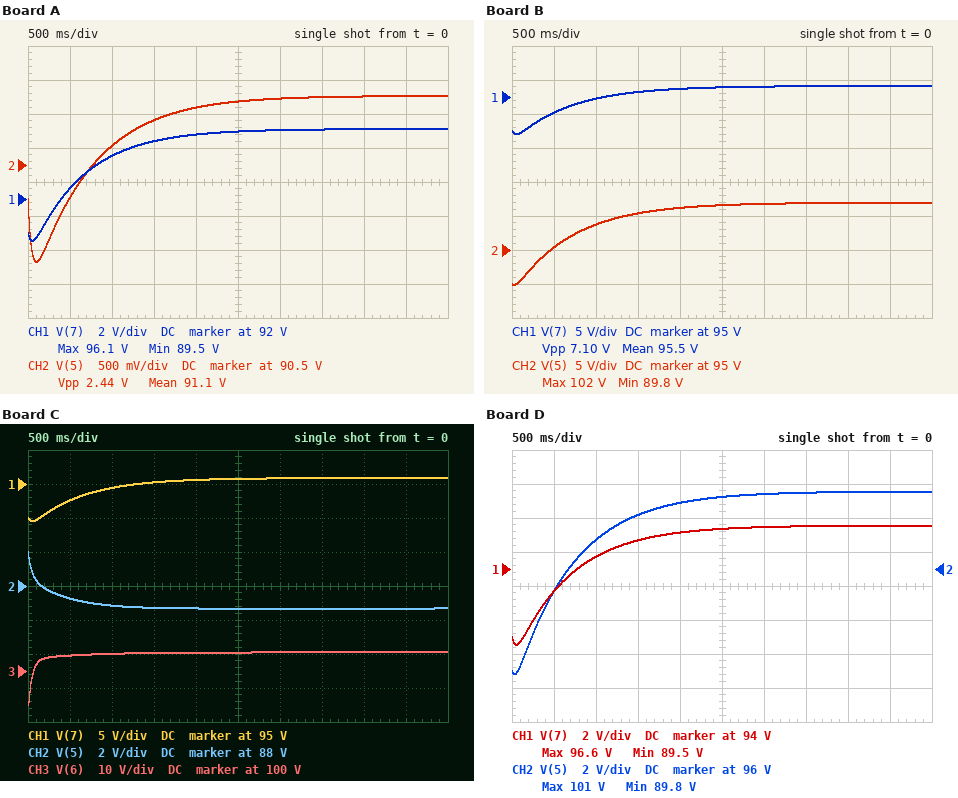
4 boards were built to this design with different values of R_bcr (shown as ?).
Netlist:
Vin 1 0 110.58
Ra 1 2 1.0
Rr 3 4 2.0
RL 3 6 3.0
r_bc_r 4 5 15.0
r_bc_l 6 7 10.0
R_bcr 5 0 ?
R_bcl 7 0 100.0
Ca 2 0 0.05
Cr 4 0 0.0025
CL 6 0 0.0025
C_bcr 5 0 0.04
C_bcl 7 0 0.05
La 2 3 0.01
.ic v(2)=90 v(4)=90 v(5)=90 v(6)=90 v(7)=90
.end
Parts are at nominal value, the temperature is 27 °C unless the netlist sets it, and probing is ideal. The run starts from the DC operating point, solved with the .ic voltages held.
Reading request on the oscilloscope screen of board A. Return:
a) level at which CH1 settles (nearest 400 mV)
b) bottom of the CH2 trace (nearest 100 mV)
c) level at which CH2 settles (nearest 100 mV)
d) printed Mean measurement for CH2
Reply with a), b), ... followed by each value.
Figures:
a) 96.0 V
b) 89.1 V
c) 91.5 V
d) 91.1 V
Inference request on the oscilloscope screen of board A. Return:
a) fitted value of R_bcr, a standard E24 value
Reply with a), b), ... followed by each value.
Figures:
a) 91 Ω
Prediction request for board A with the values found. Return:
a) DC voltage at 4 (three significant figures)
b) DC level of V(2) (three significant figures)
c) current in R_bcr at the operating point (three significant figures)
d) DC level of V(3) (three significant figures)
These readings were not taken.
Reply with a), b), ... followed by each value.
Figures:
a) 107 V
b) 109 V
c) 1.01 A
d) 109 V
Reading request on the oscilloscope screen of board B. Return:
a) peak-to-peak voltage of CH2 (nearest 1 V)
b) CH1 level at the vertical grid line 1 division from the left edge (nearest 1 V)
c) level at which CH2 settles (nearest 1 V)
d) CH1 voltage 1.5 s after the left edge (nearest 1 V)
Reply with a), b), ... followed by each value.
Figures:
a) 12 V
b) 93 V
c) 102 V
d) 96 V
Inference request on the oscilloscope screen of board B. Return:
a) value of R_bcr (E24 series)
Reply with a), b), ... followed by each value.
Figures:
a) 240 Ω
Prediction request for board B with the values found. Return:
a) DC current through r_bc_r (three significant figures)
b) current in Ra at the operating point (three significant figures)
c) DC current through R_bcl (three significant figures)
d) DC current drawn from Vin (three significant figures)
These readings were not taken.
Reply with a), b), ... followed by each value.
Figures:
a) 425 mA
b) 1.39 A
c) 966 mA
d) 1.39 A
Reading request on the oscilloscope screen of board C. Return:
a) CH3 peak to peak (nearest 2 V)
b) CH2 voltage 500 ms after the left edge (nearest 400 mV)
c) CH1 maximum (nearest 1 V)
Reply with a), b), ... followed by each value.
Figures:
a) 16 V
b) 87.2 V
c) 96 V
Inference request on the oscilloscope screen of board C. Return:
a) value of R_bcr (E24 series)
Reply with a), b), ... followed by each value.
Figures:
a) 68 Ω
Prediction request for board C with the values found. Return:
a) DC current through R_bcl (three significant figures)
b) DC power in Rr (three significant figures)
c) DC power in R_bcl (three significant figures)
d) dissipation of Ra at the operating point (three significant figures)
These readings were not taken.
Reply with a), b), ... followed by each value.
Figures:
a) 959 mA
b) 3.25 W
c) 91.9 W
d) 4.99 W
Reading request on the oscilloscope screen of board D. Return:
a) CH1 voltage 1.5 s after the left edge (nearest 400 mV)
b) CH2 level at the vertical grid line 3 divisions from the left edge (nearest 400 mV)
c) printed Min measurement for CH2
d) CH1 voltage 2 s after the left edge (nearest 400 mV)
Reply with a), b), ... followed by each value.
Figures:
a) 95.6 V
b) 99.2 V
c) 89.8 V
d) 96.0 V
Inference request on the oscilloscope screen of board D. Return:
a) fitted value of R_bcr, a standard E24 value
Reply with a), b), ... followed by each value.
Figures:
a) 200 Ω
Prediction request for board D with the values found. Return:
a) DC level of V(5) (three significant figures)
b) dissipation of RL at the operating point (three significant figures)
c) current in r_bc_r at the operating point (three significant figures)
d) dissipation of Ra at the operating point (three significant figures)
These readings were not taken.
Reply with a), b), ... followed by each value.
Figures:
a) 101 V
b) 2.80 W
c) 503 mA
d) 2.16 W
